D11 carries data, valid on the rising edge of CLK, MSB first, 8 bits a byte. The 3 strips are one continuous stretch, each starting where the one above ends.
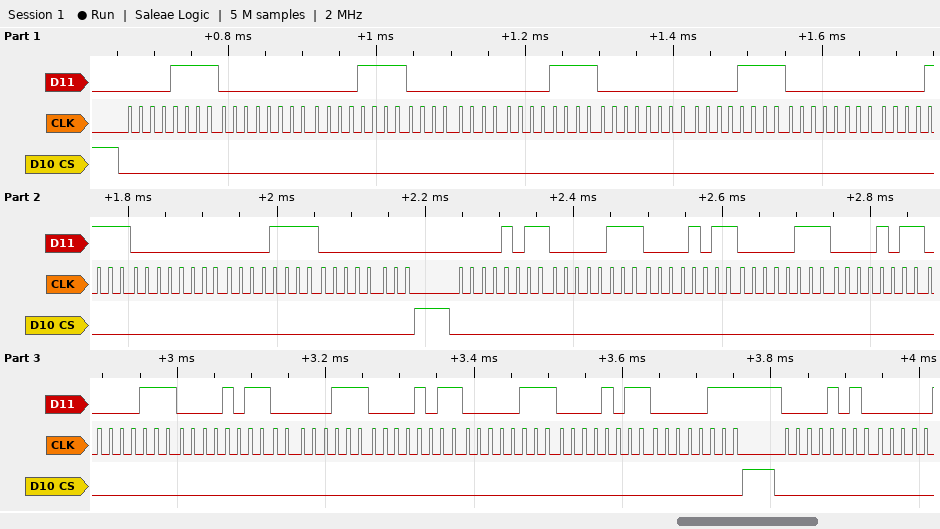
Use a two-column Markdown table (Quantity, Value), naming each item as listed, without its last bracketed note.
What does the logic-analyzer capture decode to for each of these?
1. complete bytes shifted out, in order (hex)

| Quantity | Value |
|---|---|
| complete bytes shifted out, in order | 0F 00 0F 00 0F 00 0F 00 0F 00 0F 00 0B 07 0B 07 0B 07 0B 07 0B 07 0B 07 0A |
